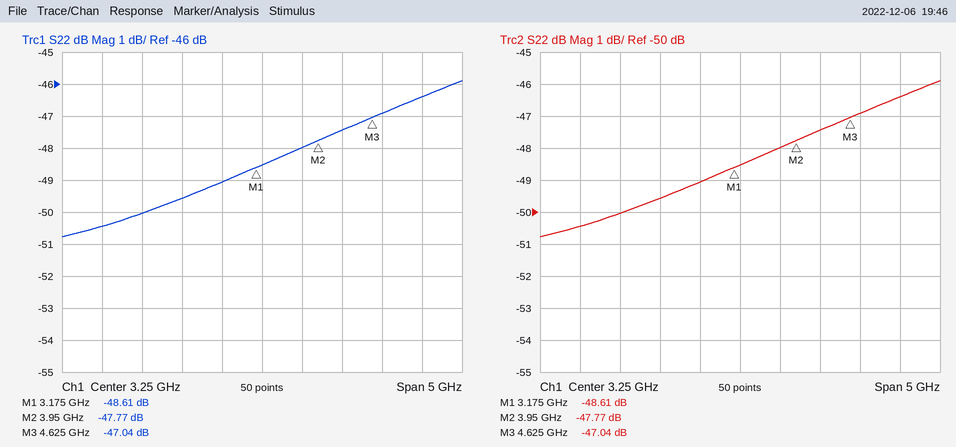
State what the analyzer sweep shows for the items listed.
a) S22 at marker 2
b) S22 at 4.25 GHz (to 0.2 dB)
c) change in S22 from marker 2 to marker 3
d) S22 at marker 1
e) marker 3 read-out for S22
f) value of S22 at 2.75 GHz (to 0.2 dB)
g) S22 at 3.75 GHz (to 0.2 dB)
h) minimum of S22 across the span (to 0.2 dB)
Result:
-47.77 dB
-47.4 dB
0.73 dB
-48.61 dB
-47.04 dB
-49.0 dB
-48.0 dB
-50.8 dB
